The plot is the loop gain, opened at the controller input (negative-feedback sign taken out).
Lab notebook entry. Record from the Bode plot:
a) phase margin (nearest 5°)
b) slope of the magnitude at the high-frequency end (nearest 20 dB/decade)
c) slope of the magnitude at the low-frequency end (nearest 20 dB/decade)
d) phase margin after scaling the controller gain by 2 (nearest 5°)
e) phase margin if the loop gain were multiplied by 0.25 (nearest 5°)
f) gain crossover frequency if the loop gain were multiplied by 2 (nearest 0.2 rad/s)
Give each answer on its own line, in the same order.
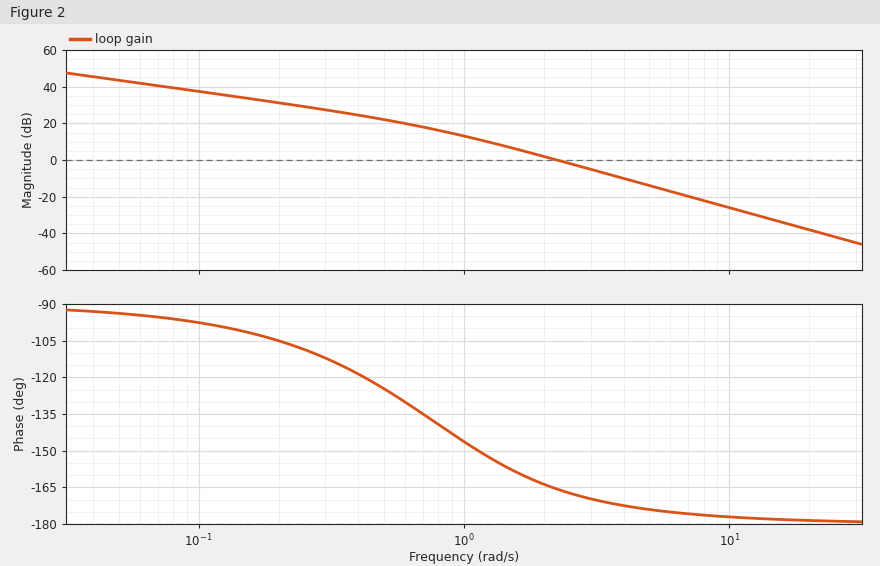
15°
-40 dB/decade
-20 dB/decade
10°
30°
3.2 rad/s
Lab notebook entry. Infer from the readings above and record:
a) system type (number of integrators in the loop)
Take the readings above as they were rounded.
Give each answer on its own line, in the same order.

1
